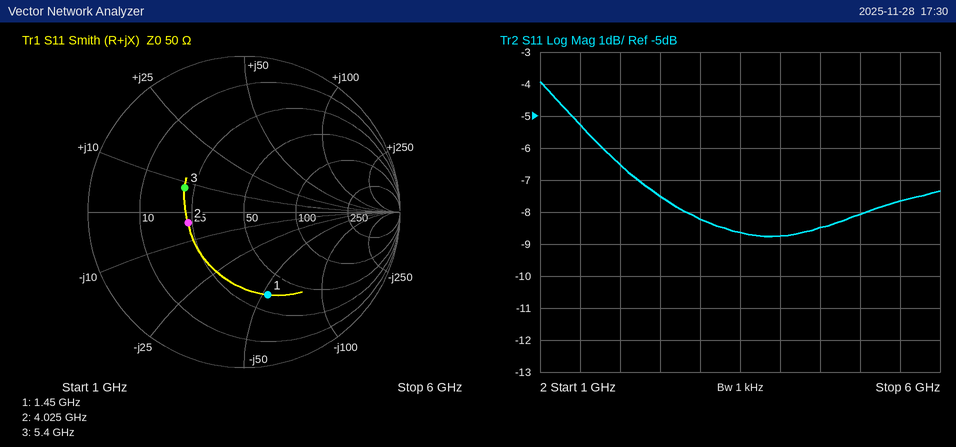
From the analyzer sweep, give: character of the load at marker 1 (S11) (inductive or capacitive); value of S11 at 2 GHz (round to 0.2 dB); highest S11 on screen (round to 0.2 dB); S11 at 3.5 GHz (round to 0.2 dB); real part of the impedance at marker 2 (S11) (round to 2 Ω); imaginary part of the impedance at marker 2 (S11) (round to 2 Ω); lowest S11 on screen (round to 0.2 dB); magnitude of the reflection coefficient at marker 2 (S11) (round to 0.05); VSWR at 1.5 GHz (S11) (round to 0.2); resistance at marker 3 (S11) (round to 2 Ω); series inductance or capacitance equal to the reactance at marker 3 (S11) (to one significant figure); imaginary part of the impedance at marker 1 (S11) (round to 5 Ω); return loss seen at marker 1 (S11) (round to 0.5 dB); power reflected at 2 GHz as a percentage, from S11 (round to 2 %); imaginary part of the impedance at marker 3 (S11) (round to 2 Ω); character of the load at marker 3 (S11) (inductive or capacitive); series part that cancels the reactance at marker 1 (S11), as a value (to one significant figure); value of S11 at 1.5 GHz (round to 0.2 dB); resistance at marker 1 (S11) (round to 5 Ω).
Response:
capacitive
-6.6 dB
-4.0 dB
-8.6 dB
24 Ω
-4 Ω
-8.8 dB
0.35
3.4
22 Ω
200 pH
-55 Ω
5.0 dB
22 %
+8 Ω
inductive
6 nH
-5.2 dB
35 Ω
